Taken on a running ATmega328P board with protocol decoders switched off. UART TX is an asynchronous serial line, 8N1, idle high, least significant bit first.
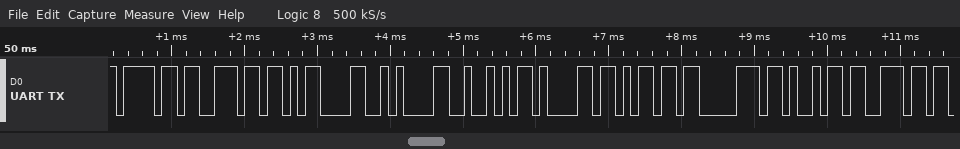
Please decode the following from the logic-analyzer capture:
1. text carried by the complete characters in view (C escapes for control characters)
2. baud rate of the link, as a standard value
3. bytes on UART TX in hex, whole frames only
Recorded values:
"on\r\nRampin"
9600 baud
6F 6E 0D 0A 52 61 6D 70 69 6E
